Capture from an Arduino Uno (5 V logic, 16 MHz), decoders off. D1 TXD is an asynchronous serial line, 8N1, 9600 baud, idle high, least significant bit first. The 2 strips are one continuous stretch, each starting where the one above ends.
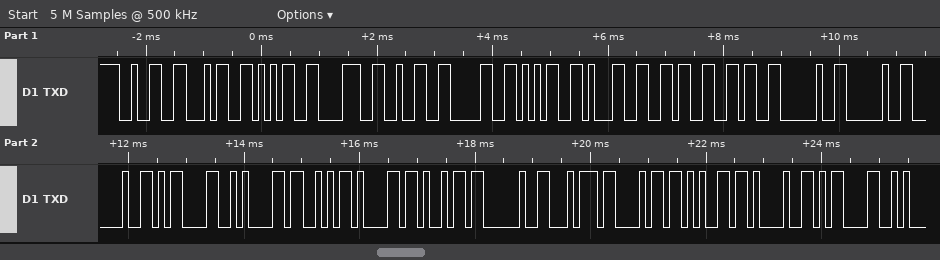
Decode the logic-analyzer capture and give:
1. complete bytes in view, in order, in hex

32 34 35 38 32 30 35 31 36 36 20 20 20 0D 0A 53 61 69 20 74 68 65 21 0D
